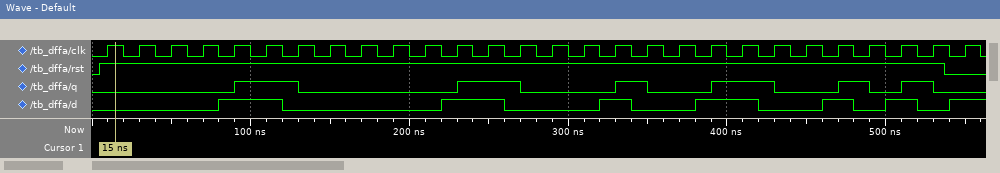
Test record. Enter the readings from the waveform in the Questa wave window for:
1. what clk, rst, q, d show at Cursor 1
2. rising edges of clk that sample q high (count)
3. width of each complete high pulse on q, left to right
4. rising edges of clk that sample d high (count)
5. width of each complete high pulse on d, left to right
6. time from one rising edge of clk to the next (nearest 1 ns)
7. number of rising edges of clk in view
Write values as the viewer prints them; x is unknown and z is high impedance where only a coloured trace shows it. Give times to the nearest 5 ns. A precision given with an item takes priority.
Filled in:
clk=1, rst=1, q=0, d=0
9
40 ns, 40 ns, 20 ns, 40 ns, 20 ns, 20 ns
10
40 ns, 40 ns, 20 ns, 40 ns, 20 ns, 20 ns
20 ns
28
